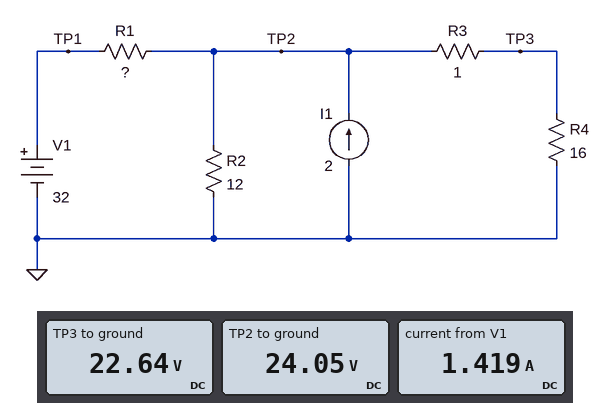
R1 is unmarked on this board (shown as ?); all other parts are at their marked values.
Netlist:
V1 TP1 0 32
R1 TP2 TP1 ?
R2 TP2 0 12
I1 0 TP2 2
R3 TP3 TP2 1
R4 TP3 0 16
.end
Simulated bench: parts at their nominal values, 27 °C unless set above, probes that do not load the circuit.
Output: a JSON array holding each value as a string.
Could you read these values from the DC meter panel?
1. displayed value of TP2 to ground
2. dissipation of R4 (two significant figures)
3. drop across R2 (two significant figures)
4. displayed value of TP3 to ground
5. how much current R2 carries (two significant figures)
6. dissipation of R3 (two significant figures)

["24.05 V", "32 W", "24 V", "22.64 V", "2.0 A", "2.0 W"]
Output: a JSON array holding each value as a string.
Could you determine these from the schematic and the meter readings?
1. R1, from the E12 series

["5.6 Ω"]
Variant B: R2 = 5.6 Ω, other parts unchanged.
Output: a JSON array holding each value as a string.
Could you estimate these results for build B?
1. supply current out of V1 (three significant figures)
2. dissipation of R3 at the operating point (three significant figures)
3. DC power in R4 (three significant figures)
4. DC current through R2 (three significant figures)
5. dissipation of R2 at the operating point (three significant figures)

["2.40 A", "1.19 W", "19.0 W", "3.31 A", "61.4 W"]
